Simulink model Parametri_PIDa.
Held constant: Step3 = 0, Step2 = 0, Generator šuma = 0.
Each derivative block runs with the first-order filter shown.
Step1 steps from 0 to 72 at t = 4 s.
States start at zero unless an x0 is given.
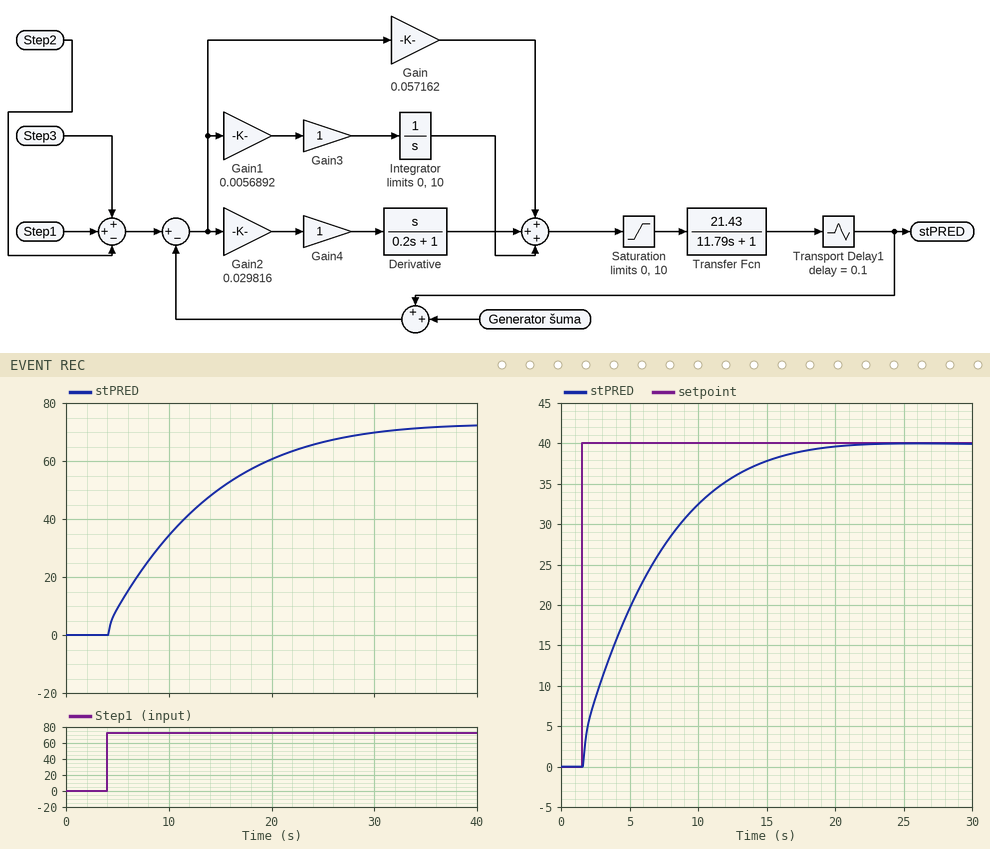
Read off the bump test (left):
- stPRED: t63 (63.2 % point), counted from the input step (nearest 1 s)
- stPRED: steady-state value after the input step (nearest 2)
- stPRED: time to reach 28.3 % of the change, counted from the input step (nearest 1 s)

9 s
72
3 s
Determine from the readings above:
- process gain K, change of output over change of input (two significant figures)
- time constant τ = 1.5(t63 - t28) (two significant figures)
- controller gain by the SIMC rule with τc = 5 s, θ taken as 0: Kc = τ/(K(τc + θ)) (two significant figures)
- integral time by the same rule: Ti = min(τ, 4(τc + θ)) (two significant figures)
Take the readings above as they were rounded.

1.0
9.0 s
1.8
9.0 s
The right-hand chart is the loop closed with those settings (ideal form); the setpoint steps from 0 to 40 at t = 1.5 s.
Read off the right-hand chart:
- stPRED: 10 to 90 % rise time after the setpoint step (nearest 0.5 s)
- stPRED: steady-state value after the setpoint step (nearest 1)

11.0 s
40
